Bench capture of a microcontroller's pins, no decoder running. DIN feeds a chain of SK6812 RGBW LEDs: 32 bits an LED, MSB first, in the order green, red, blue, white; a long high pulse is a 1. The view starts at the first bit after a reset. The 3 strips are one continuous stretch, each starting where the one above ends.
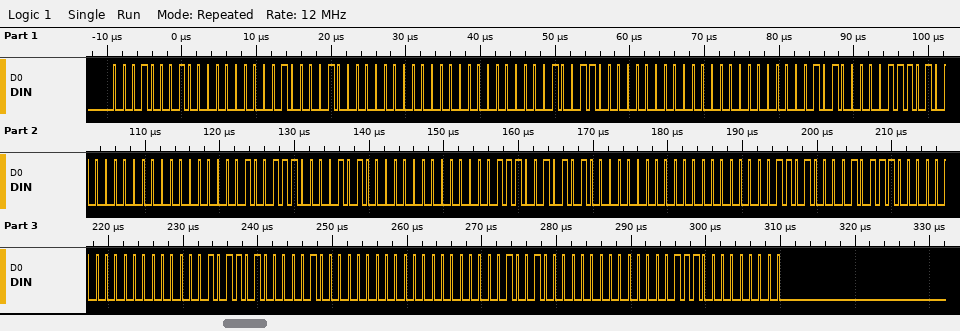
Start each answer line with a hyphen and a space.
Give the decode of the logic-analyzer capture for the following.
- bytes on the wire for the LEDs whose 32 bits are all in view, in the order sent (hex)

- 11 00 21 00 00 01 30 00 00 14 1D 00 00 27 0A 00 07 2A 00 00 1A 17 00 00 2D 04 00 00 24 00 0E 00
